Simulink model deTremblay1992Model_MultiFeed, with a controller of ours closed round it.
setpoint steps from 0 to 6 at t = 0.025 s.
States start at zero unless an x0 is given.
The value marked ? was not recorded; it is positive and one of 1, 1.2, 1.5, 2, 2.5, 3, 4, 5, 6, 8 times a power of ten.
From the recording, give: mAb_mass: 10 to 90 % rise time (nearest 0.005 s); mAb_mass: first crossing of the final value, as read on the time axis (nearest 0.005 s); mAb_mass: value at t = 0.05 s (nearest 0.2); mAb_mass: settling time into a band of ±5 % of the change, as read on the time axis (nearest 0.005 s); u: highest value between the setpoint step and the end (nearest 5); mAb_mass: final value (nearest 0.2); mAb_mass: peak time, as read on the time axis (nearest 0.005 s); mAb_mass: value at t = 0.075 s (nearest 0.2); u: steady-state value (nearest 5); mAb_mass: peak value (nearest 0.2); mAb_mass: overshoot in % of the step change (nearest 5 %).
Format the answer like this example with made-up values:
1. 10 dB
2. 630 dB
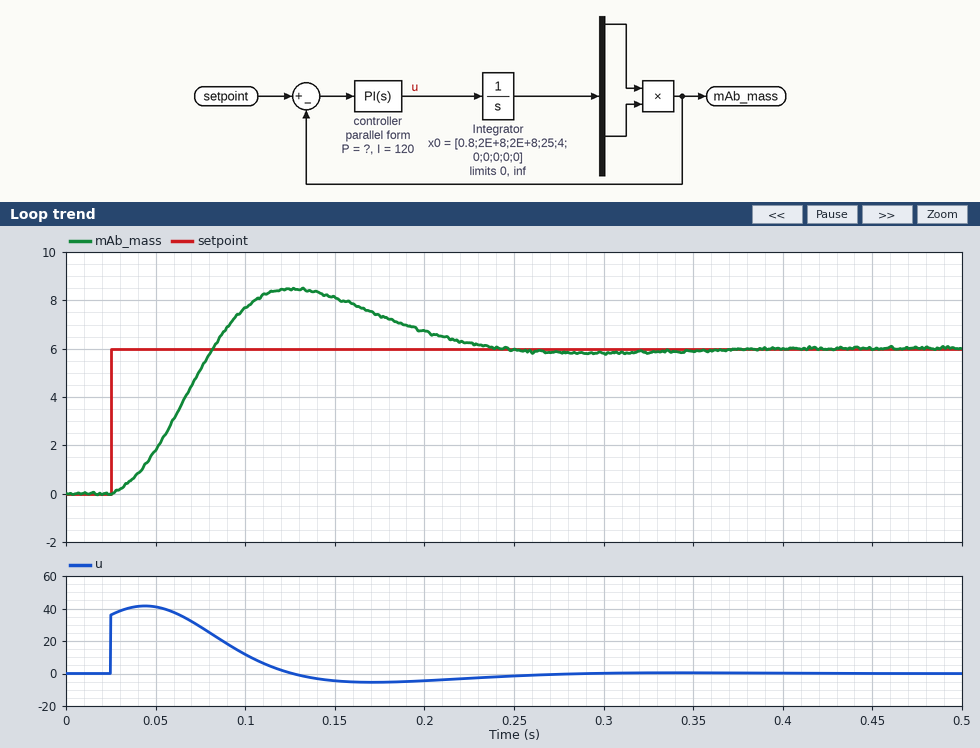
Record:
1. 0.040 s
2. 0.080 s
3. 1.8
4. 0.220 s
5. 40
6. 6.0
7. 0.125 s
8. 5.2
9. 0
10. 8.4
11. 40 %
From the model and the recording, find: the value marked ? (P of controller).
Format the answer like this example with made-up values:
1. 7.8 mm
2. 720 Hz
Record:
1. 6
